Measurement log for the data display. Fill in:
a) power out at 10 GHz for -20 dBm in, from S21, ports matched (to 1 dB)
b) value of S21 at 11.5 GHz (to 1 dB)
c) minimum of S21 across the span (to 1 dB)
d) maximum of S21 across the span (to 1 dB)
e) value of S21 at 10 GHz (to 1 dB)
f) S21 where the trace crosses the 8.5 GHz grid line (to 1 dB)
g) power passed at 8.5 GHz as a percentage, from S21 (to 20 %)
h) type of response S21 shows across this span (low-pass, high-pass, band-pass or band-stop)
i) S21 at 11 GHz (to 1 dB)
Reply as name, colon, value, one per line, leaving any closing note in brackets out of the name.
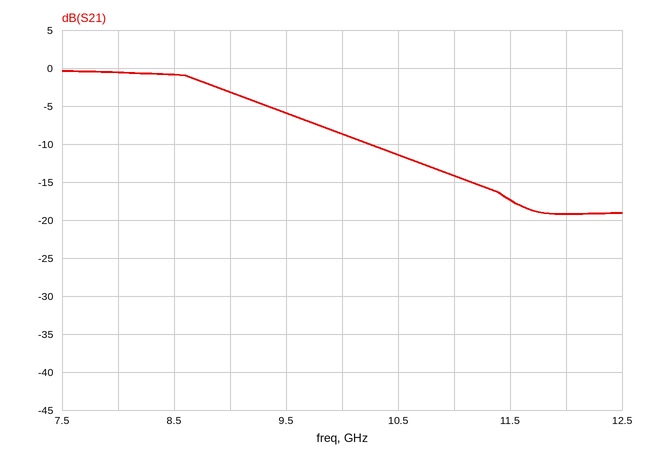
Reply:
power out at 10 GHz for -20 dBm in, from S21, ports matched: -29 dBm
value of S21 at 11.5 GHz: -17 dB
minimum of S21 across the span: -19 dB
maximum of S21 across the span: 0 dB
value of S21 at 10 GHz: -9 dB
S21 where the trace crosses the 8.5 GHz grid line: -1 dB
power passed at 8.5 GHz as a percentage, from S21: 80 %
type of response S21 shows across this span: low-pass
S21 at 11 GHz: -14 dB
